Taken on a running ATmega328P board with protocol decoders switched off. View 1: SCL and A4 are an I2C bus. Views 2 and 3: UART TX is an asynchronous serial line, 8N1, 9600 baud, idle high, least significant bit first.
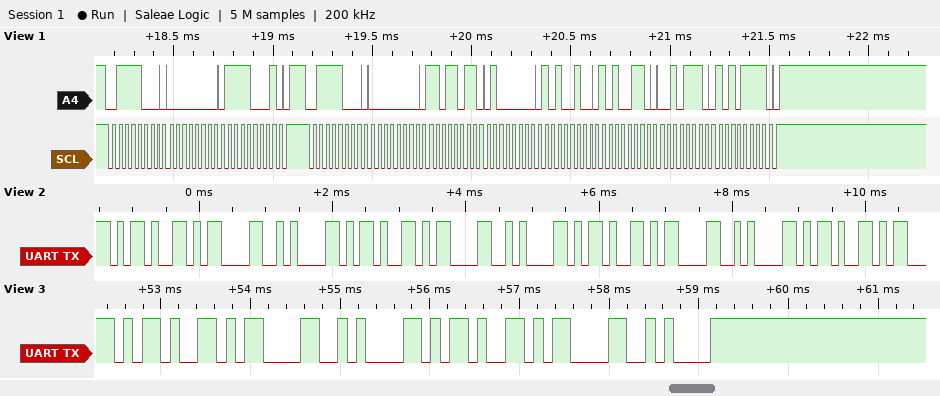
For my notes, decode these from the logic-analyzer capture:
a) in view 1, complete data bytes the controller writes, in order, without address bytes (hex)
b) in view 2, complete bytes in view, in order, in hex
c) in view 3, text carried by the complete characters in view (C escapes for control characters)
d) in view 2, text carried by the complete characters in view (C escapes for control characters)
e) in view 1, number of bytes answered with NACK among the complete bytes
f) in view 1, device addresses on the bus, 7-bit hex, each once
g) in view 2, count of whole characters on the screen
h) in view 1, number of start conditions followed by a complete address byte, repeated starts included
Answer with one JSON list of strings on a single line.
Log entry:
["00 F1 00 DB 40 A4 A6 2E AF", "2D 0D 0A 2D 0D 0A 2D 0D 0A 2D", "\"-\\r\\n-\\r\\n\"", "\"-\\r\\n-\\r\\n-\\r\\n-\"", "0", "0x3C", "10", "2"]
